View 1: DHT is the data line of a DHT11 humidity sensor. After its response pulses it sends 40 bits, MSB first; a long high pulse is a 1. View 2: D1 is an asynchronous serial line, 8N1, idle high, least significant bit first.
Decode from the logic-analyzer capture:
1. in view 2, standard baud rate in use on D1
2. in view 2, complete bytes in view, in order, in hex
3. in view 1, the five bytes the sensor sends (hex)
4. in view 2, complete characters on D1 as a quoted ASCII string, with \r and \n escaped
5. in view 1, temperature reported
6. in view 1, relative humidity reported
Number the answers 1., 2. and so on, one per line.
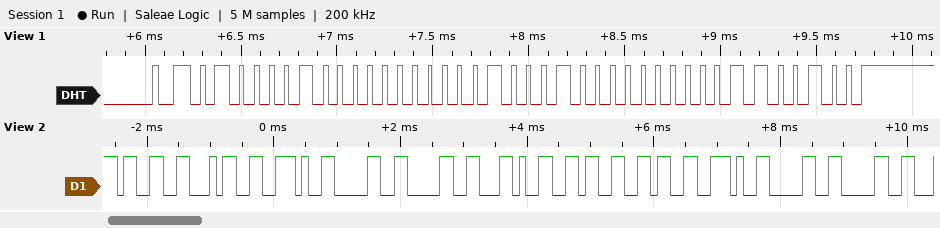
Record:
1. 9600 baud
2. 33 34 2E 30 30 2C 36 36 2E 30 30
3. 42 00 22 00 64
4. "34.00,66.00"
5. 34.0 °C
6. 66 %
